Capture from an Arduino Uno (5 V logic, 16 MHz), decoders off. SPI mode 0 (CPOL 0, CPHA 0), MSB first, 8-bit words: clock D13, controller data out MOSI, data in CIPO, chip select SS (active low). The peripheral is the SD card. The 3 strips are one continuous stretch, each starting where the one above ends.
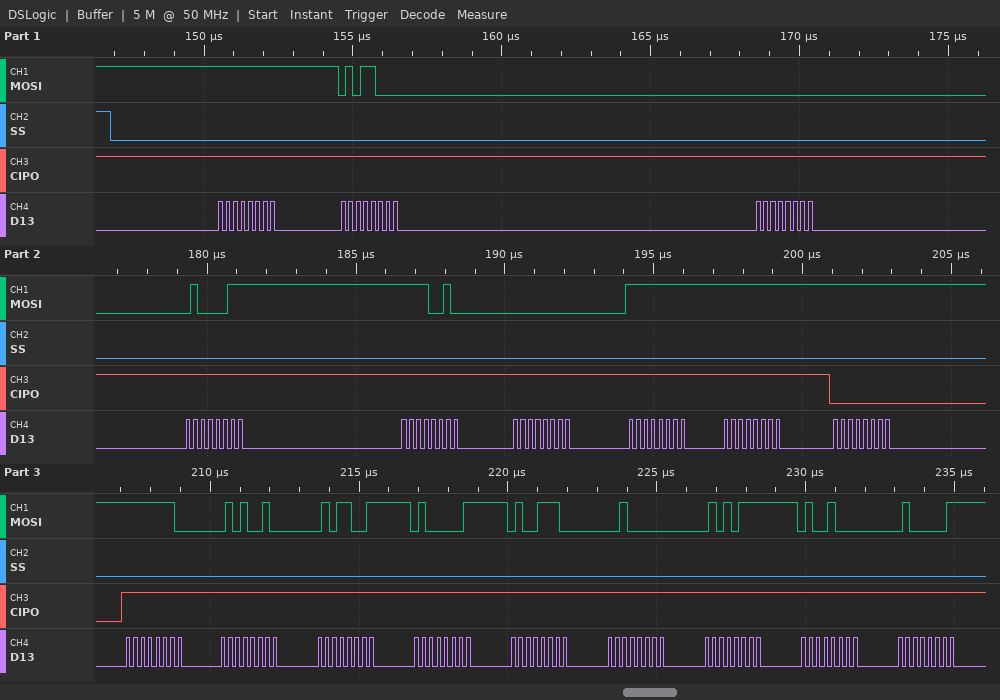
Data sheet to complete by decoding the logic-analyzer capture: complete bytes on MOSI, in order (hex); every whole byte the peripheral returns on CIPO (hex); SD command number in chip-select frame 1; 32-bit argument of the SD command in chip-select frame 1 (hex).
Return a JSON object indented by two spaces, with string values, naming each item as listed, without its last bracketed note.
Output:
{
  "complete bytes on MOSI, in order": "FF 58 00 43 F2 00 FF FF FF FE 52 59 41 4E 20 57 48 41",
  "every whole byte the peripheral returns on CIPO": "FF FF FF FF FF FF FF FF 00 FF FF FF FF FF FF FF FF FF",
  "SD command number in chip-select frame 1": "CMD24",
  "32-bit argument of the SD command in chip-select frame 1": "0x0043F200"
}
